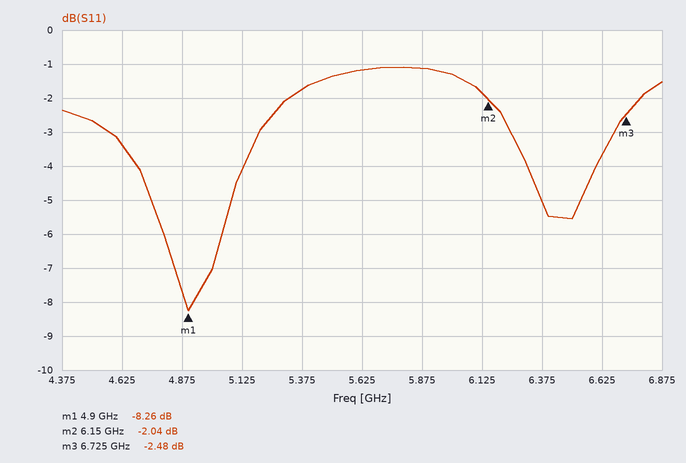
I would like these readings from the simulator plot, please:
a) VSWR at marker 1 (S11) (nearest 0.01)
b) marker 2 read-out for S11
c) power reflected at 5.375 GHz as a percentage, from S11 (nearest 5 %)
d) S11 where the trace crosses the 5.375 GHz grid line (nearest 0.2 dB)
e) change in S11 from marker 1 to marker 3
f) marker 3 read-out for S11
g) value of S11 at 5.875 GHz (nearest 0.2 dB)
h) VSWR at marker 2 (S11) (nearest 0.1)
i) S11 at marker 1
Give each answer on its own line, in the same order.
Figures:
2.26
-2.04 dB
65 %
-1.8 dB
5.78 dB
-2.48 dB
-1.2 dB
8.6
-8.26 dB
